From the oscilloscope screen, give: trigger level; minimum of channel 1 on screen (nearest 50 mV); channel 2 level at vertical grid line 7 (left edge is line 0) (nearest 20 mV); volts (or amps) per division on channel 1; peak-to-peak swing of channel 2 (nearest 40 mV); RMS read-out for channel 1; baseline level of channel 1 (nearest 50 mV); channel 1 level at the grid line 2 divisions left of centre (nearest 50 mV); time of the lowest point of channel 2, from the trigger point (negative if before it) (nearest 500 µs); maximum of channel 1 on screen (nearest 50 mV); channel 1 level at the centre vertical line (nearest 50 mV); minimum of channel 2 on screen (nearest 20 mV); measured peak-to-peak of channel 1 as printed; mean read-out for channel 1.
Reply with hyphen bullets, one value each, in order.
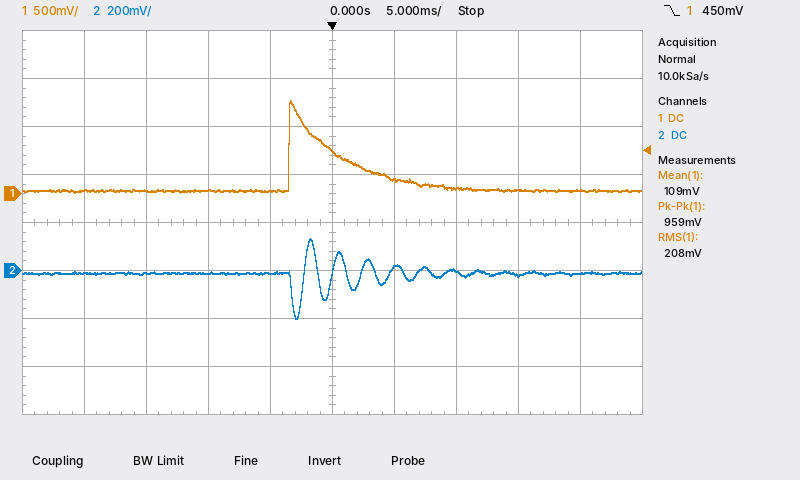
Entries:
- 450 mV
- 0 mV
- 0 mV
- 500 mV
- 320 mV
- 208 mV
- 50 mV
- 50 mV
- -3.0 ms
- 950 mV
- 450 mV
- -200 mV
- 959 mV
- 109 mV
